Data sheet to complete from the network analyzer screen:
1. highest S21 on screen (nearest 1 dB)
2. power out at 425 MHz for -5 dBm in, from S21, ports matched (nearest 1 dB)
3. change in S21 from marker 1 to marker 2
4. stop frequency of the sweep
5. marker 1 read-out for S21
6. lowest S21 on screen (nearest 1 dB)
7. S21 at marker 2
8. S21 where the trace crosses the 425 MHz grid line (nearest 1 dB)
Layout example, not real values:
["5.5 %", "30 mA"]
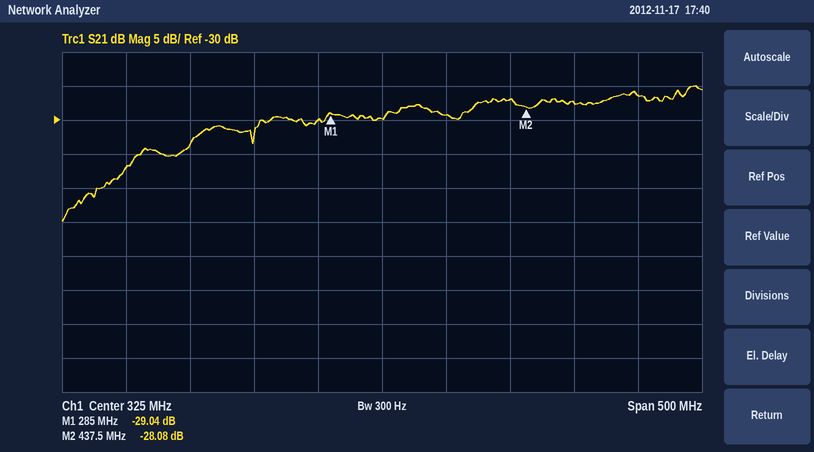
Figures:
["-25 dB", "-32 dBm", "0.96 dB", "575 MHz", "-29.04 dB", "-45 dB", "-28.08 dB", "-27 dB"]
